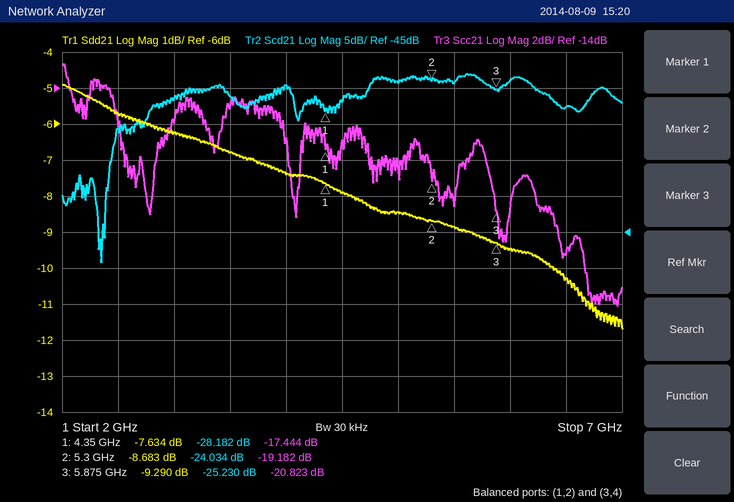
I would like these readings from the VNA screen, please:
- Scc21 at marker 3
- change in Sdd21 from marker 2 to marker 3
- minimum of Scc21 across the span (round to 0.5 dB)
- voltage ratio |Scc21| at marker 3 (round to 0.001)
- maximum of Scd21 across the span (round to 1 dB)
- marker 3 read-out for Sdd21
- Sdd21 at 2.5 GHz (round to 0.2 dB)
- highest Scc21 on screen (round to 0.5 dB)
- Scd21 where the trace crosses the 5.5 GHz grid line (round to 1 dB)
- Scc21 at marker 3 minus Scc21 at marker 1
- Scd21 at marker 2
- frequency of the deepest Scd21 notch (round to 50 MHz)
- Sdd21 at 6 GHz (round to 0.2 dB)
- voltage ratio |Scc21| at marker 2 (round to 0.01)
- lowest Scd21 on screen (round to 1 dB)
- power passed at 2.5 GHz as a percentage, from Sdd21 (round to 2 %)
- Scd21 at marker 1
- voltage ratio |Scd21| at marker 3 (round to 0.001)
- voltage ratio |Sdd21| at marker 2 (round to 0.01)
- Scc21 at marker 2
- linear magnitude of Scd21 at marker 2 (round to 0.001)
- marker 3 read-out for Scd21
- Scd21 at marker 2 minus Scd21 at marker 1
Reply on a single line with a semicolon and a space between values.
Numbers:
-20.823 dB; -0.607 dB; -26.0 dB; 0.091; -23 dB; -9.290 dB; -5.8 dB; -12.5 dB; -24 dB; -3.379 dB; -24.034 dB; 2.35 GHz; -9.4 dB; 0.11; -49 dB; 26 %; -28.182 dB; 0.055; 0.37; -19.182 dB; 0.063; -25.230 dB; 4.148 dB
